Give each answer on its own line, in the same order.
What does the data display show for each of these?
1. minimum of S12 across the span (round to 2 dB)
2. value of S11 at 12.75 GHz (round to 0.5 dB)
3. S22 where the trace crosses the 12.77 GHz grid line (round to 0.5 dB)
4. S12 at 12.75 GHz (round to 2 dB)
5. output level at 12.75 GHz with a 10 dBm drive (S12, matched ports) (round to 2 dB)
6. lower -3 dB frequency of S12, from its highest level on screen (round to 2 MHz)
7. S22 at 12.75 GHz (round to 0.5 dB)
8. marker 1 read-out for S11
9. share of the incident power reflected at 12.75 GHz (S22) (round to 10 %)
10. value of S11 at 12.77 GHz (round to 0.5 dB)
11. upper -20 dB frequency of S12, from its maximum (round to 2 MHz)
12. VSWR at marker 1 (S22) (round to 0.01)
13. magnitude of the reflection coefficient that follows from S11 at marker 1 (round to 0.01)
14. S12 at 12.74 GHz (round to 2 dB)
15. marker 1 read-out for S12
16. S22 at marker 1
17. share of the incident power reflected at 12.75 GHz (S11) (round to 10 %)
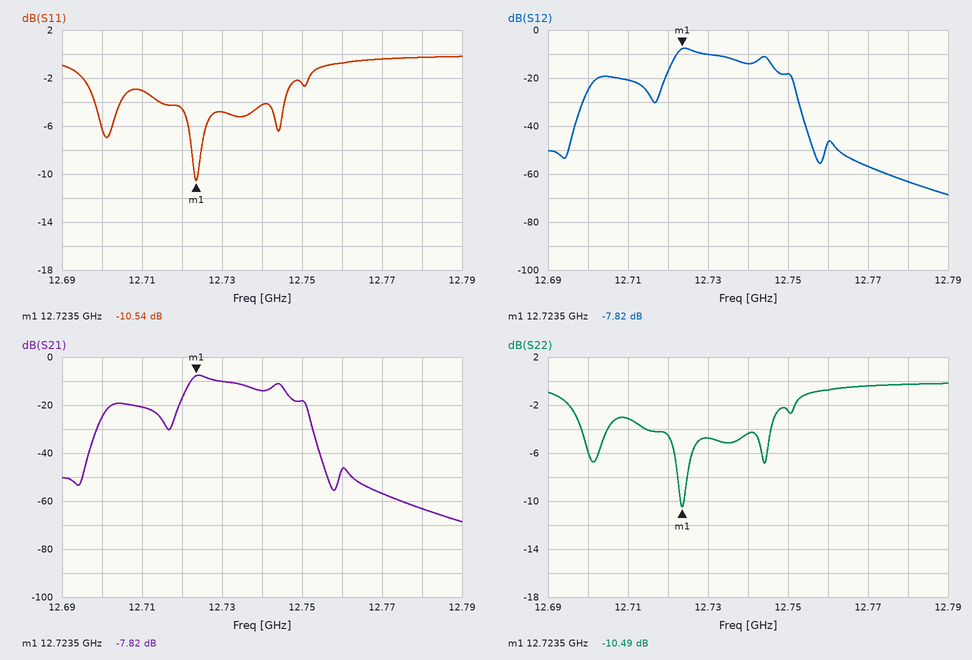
-68 dB
-2.5 dB
-0.5 dB
-18 dB
-8 dBm
12.722 GHz
-2.5 dB
-10.54 dB
60 %
-0.5 dB
12.752 GHz
1.85
0.30
-14 dB
-7.82 dB
-10.49 dB
60 %
